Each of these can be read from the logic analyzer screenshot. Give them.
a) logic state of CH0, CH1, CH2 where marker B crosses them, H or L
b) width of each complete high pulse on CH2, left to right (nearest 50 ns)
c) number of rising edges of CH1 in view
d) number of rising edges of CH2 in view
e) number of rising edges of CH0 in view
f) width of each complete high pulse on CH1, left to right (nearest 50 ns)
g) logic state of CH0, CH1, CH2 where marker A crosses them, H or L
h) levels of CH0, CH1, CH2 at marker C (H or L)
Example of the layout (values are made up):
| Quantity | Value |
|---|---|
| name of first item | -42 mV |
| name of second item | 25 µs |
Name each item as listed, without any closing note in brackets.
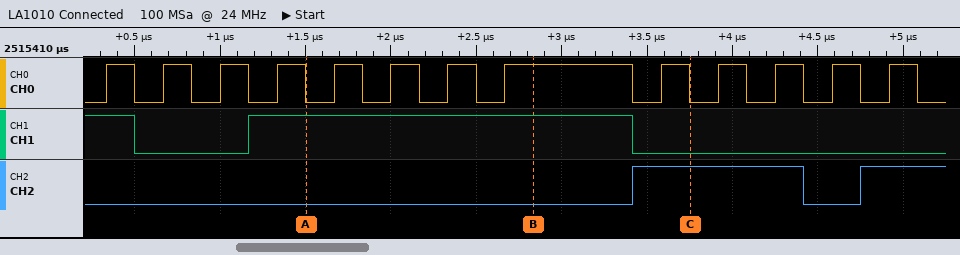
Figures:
| Quantity | Value |
|---|---|
| logic state of CH0, CH1, CH2 where marker B crosses them, H or L | CH0=H, CH1=H, CH2=L |
| width of each complete high pulse on CH2, left to right | 1000 ns |
| number of rising edges of CH1 in view | 1 |
| number of rising edges of CH2 in view | 2 |
| number of rising edges of CH0 in view | 13 |
| width of each complete high pulse on CH1, left to right | 2250 ns |
| logic state of CH0, CH1, CH2 where marker A crosses them, H or L | CH0=L, CH1=H, CH2=L |
| levels of CH0, CH1, CH2 at marker C | CH0=L, CH1=L, CH2=H |
